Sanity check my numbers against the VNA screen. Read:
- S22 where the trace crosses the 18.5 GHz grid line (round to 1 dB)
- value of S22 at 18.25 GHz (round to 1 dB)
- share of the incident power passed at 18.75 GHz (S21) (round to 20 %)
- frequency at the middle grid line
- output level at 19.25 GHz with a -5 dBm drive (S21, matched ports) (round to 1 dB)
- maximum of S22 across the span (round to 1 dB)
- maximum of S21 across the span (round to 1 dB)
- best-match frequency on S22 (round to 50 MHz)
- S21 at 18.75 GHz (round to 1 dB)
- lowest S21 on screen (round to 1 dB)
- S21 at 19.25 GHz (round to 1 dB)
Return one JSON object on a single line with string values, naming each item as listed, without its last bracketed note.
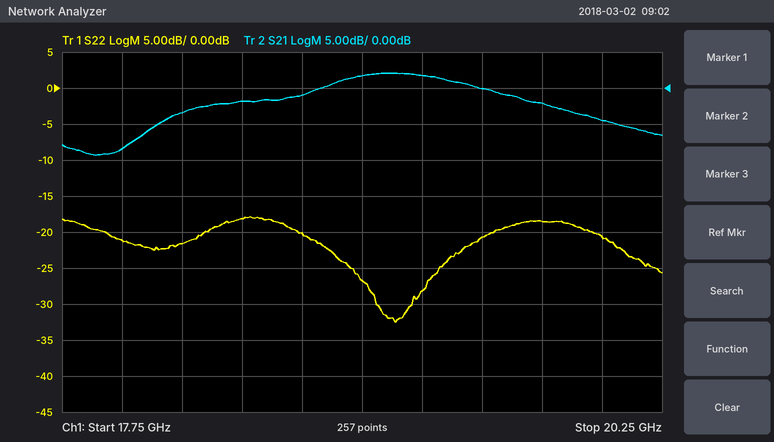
{"S22 where the trace crosses the 18.5 GHz grid line": "-18 dB", "value of S22 at 18.25 GHz": "-22 dB", "share of the incident power passed at 18.75 GHz (S21)": "80 %", "frequency at the middle grid line": "19 GHz", "output level at 19.25 GHz with a -5 dBm drive (S21, matched ports)": "-3 dBm", "maximum of S22 across the span": "-18 dB", "maximum of S21 across the span": "2 dB", "best-match frequency on S22": "19.15 GHz", "S21 at 18.75 GHz": "-1 dB", "lowest S21 on screen": "-9 dB", "S21 at 19.25 GHz": "2 dB"}
